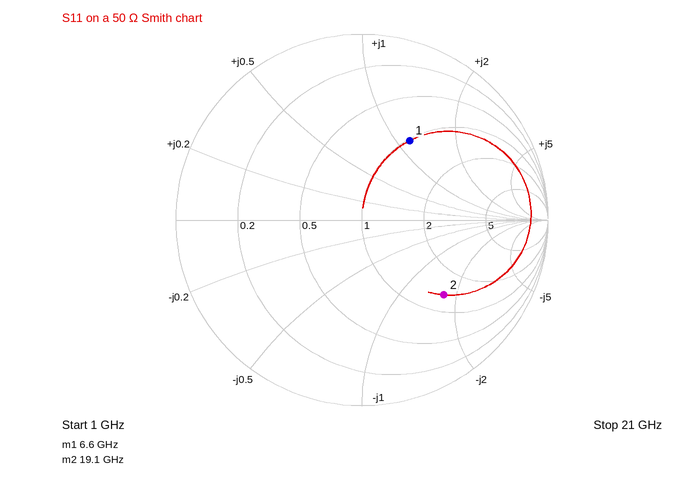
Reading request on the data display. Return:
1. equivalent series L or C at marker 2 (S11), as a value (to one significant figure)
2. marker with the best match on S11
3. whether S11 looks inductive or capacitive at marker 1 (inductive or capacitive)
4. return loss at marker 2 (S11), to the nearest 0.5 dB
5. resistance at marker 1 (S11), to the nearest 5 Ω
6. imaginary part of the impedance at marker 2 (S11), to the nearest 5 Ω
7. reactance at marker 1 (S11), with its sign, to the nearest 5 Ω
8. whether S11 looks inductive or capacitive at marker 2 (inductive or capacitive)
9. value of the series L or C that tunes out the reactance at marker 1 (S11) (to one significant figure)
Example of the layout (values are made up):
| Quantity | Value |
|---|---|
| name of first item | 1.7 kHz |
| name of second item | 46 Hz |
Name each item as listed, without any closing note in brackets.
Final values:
| Quantity | Value |
|---|---|
| equivalent series L or C at marker 2 (S11), as a value | 100 fF |
| marker with the best match on S11 | marker 1 |
| whether S11 looks inductive or capacitive at marker 1 | inductive |
| return loss at marker 2 (S11), to the nearest 0.5 dB | 4.5 dB |
| resistance at marker 1 (S11), to the nearest 5 Ω | 50 Ω |
| imaginary part of the impedance at marker 2 (S11), to the nearest 5 Ω | -85 Ω |
| reactance at marker 1 (S11), with its sign, to the nearest 5 Ω | +60 Ω |
| whether S11 looks inductive or capacitive at marker 2 | capacitive |
| value of the series L or C that tunes out the reactance at marker 1 (S11) | 400 fF |
